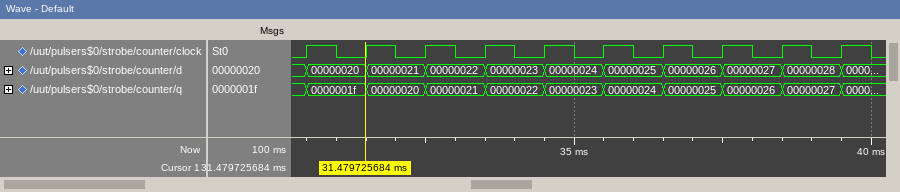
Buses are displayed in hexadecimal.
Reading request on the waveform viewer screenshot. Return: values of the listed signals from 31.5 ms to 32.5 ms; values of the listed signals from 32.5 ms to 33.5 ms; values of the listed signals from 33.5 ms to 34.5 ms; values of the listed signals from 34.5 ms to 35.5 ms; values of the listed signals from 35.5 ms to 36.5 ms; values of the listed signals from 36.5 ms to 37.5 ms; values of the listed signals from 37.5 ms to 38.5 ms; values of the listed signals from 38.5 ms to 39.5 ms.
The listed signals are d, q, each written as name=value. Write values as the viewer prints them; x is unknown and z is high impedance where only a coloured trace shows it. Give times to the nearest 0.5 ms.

d=00000021, q=00000020
d=00000022, q=00000021
d=00000023, q=00000022
d=00000024, q=00000023
d=00000025, q=00000024
d=00000026, q=00000025
d=00000027, q=00000026
d=00000028, q=00000027
